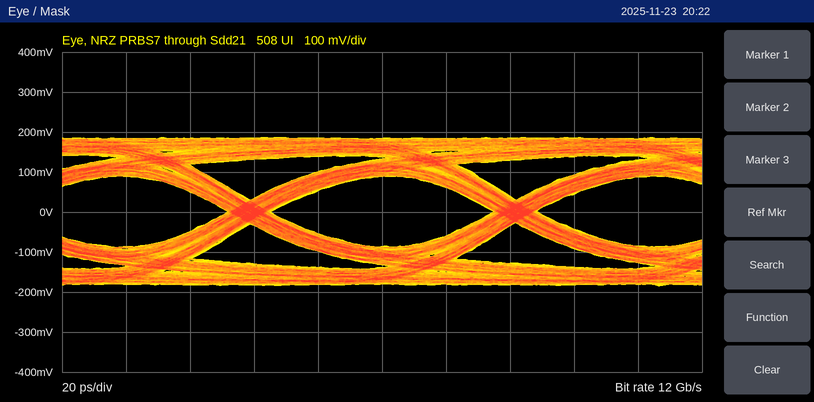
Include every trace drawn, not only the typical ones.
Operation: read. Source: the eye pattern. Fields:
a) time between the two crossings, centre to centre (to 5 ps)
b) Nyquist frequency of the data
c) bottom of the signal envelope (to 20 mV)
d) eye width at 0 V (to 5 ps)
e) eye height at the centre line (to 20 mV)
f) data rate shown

85 ps
6 GHz
-180 mV
70 ps
180 mV
12 Gb/s
